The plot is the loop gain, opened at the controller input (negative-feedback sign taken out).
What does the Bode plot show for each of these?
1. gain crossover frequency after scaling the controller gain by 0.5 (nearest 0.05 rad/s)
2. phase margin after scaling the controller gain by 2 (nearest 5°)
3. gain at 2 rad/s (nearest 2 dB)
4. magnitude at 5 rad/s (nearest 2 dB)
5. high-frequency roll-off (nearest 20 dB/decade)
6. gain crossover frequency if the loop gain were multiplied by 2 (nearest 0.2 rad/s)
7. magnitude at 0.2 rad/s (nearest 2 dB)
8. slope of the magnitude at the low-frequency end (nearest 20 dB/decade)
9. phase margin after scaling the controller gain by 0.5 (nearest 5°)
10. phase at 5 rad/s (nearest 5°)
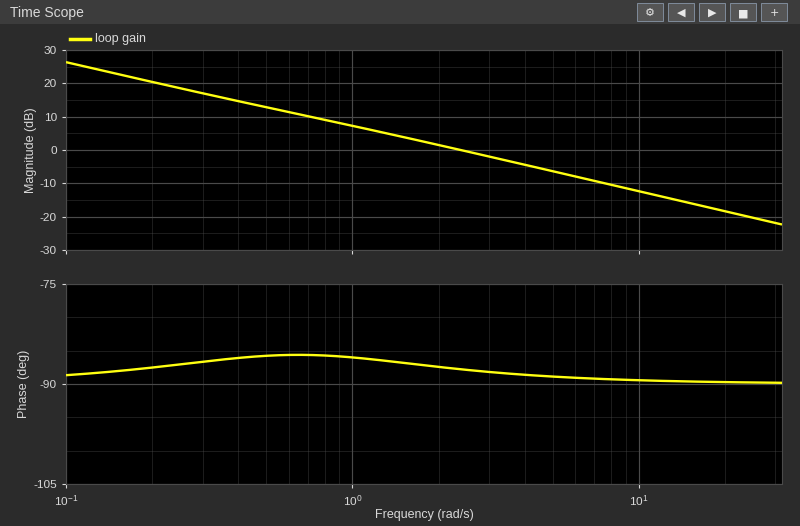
1.15 rad/s
90°
2 dB
-6 dB
-20 dB/decade
4.8 rad/s
20 dB
-20 dB/decade
95°
-90°
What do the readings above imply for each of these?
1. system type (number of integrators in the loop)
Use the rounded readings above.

1
